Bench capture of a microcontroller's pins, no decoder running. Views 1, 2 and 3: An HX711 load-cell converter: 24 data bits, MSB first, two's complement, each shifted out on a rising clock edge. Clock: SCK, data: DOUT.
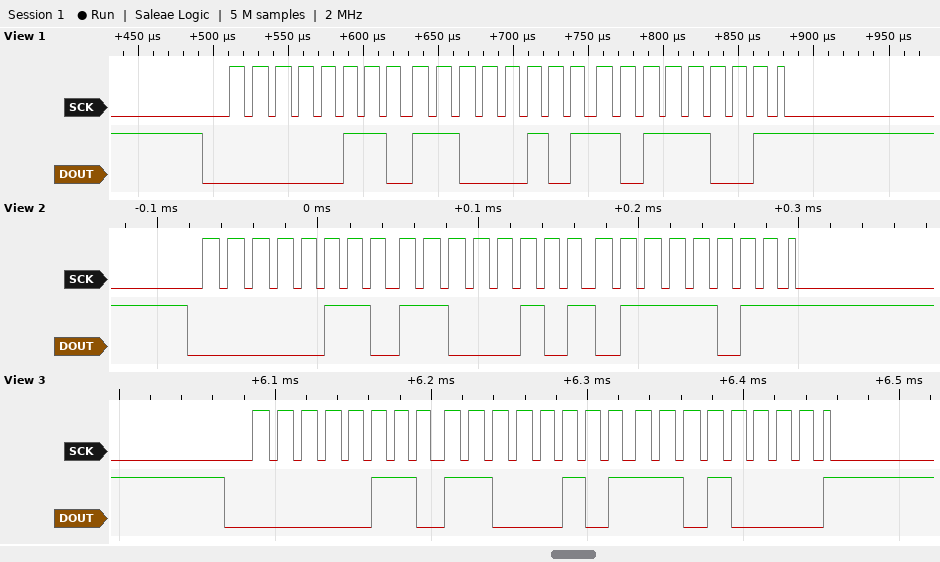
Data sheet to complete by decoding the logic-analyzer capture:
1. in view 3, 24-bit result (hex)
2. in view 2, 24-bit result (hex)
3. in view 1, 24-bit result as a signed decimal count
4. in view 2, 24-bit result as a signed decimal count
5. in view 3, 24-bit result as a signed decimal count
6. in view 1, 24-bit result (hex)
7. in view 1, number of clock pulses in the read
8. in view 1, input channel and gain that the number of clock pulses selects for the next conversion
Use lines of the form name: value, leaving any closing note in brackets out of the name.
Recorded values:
in view 3, 24-bit result: 0x06C5D0
in view 2, 24-bit result: 0x06C57B
in view 1, 24-bit result as a signed decimal count: 443833
in view 2, 24-bit result as a signed decimal count: 443771
in view 3, 24-bit result as a signed decimal count: 443856
in view 1, 24-bit result: 0x06C5B9
in view 1, number of clock pulses in the read: 25
in view 1, input channel and gain that the number of clock pulses selects for the next conversion: channel A, gain 128
